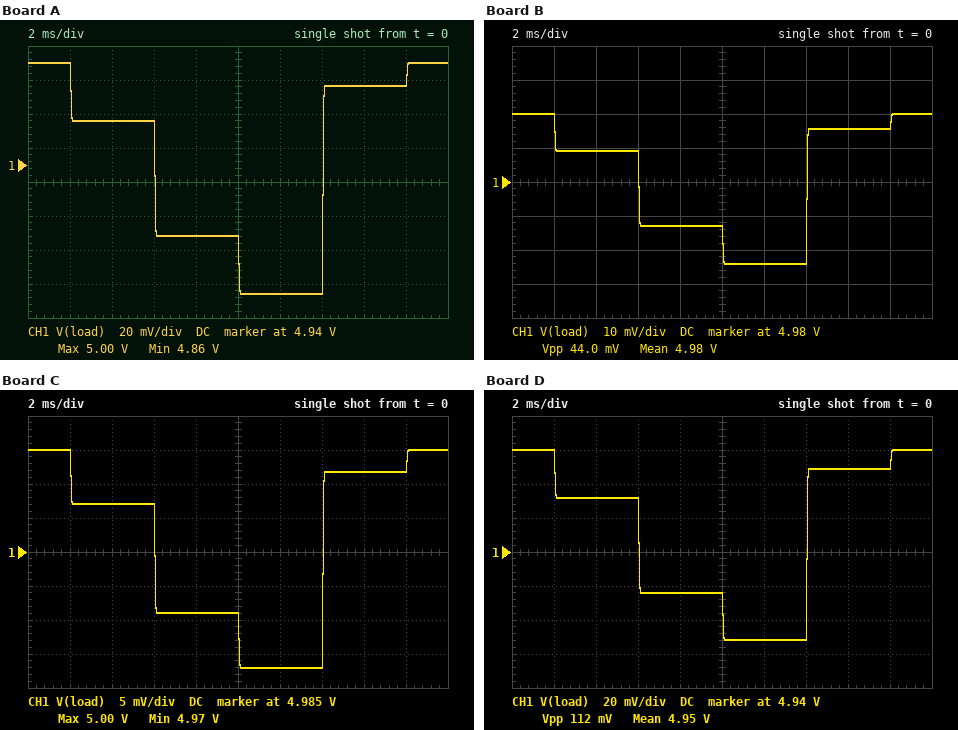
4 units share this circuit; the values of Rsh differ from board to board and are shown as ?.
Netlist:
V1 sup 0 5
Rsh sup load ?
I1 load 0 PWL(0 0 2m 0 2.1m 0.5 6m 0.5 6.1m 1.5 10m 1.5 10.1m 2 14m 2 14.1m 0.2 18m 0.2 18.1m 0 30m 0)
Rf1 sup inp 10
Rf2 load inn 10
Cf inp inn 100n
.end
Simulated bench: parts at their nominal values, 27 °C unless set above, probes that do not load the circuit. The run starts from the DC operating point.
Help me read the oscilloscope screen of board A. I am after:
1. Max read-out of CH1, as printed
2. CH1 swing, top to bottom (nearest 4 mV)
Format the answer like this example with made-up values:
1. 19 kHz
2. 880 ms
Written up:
1. 5.00 V
2. 136 mV
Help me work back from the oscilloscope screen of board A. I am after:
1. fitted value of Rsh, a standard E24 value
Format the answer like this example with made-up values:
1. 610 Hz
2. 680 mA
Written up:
1. 0.068 Ω
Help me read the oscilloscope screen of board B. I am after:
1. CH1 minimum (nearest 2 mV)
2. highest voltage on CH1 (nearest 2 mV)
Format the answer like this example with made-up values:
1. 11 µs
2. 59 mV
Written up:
1. 4.956 V
2. 5.000 V
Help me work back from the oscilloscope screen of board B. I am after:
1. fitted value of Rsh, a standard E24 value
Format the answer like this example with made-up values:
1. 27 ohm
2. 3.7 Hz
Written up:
1. 0.022 Ω
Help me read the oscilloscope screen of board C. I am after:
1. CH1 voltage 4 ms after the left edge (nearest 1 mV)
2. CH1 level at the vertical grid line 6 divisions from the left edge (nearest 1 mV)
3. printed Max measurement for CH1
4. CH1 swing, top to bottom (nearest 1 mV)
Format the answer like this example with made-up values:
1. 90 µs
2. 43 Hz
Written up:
1. 4.992 V
2. 4.968 V
3. 5.00 V
4. 32 mV
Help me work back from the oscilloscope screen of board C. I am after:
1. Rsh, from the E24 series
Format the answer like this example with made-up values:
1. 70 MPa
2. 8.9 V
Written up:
1. 0.016 Ω
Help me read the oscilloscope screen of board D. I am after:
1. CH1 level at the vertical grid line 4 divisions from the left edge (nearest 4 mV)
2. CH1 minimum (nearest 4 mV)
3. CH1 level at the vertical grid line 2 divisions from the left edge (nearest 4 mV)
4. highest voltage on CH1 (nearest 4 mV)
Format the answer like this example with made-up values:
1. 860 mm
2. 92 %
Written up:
1. 4.916 V
2. 4.888 V
3. 4.972 V
4. 5.000 V
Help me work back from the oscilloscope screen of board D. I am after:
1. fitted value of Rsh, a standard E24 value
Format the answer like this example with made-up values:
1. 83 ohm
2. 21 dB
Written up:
1. 0.056 Ω
